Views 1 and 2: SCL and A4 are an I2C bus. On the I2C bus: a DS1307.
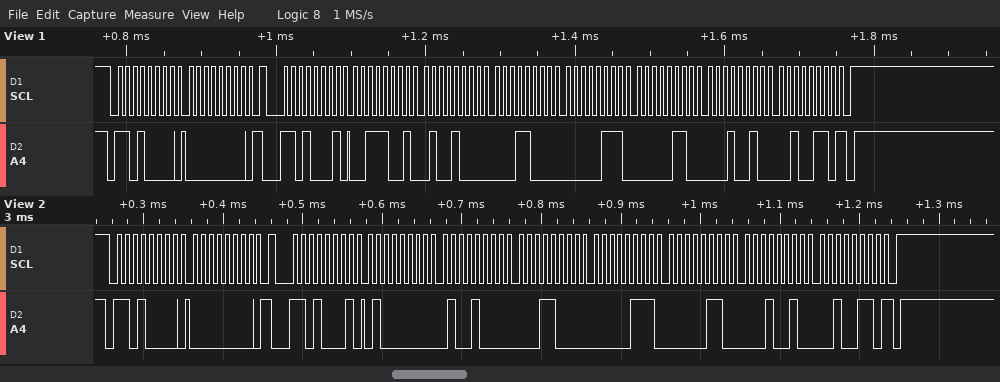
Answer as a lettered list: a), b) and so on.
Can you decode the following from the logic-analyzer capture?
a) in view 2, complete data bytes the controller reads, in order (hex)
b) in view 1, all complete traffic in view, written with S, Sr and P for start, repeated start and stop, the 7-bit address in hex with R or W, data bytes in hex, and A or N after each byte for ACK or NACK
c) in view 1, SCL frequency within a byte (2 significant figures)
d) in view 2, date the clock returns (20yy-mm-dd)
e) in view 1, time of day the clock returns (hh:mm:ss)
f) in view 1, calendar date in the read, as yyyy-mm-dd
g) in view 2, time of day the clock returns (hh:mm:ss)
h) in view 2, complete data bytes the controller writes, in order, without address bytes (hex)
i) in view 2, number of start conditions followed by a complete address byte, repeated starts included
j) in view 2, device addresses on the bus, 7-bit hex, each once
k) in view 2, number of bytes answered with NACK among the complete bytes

a) 40 48 18 07 06 12 26
b) S 68W A 00 A Sr 68R A 39 A 48 A 18 A 07 A 06 A 12 A 26 N P
c) 100 kHz
d) 2026-12-06
e) 18:48:39
f) 2026-12-06
g) 18:48:40
h) 00
i) 2
j) 0x68
k) 1
